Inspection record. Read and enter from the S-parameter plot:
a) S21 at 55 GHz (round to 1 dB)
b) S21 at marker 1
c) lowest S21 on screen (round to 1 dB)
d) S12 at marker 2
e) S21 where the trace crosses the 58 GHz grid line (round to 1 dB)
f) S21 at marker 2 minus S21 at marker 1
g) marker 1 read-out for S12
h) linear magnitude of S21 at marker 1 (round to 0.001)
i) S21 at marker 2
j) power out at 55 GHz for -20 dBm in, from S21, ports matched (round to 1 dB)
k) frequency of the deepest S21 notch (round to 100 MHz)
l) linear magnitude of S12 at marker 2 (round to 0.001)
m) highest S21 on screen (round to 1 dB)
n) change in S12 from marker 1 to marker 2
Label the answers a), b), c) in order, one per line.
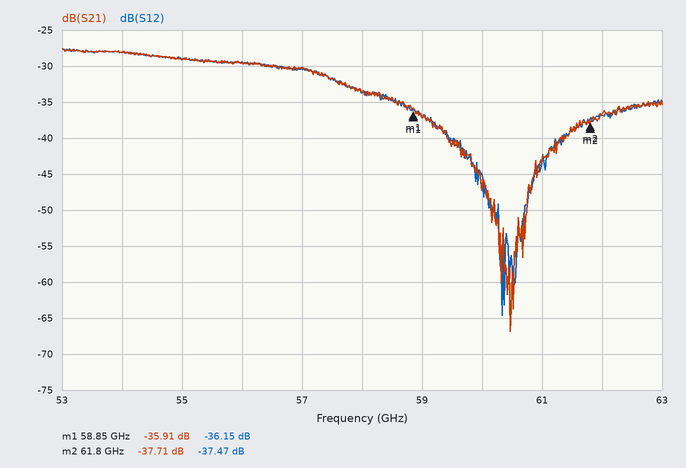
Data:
a) -29 dB
b) -35.91 dB
c) -67 dB
d) -37.47 dB
e) -34 dB
f) -1.80 dB
g) -36.15 dB
h) 0.016
i) -37.71 dB
j) -49 dBm
k) 60.5 GHz
l) 0.013
m) -28 dB
n) -1.32 dB
